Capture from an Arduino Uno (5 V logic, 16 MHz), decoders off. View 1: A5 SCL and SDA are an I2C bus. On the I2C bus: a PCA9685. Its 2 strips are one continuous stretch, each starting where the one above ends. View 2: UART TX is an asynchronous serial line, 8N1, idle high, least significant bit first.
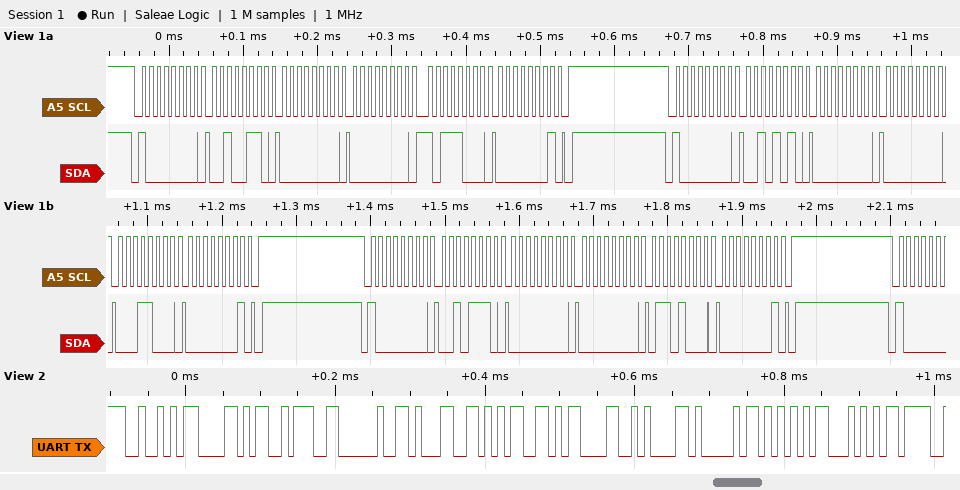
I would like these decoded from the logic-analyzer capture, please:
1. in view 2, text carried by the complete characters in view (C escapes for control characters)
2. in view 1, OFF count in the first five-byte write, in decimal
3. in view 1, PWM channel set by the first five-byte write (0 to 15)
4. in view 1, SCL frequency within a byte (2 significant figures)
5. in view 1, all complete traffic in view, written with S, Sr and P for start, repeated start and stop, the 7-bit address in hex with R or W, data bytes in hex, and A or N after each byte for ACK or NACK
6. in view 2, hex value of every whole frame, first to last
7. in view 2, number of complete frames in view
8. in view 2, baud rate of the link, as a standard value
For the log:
"RX: 15\r\nAUT"
440
8
100 kHz
S 40W A 26 A 00 A 00 A B8 A 01 A P S 40W A 2A A 00 A 00 A 18 A 01 A P S 40W A 2E A 00 A 00 A 68 A 01 A P
52 58 3A 20 31 35 0D 0A 41 55 54
11
115200 baud
